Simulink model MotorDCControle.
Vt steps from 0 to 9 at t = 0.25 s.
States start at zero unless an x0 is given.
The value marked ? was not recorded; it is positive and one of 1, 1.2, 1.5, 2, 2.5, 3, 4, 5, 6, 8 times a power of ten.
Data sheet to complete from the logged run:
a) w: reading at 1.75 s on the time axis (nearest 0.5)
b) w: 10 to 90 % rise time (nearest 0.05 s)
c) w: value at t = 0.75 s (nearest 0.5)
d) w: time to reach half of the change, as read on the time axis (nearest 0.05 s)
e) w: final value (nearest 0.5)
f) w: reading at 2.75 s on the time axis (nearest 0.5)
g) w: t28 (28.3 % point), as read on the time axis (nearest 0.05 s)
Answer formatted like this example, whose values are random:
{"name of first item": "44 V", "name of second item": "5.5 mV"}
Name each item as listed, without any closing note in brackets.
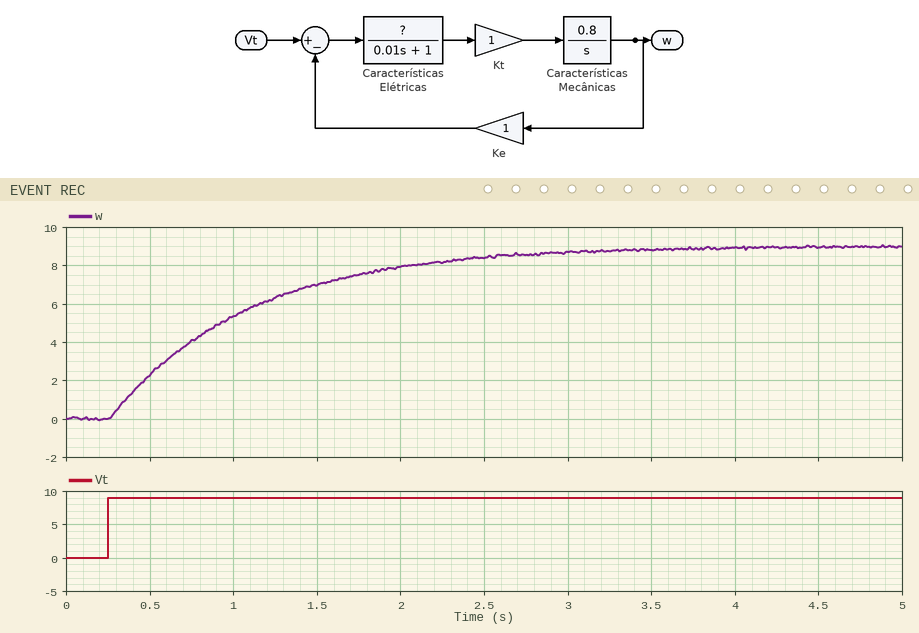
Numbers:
{"w: reading at 1.75 s on the time axis": "7.5", "w: 10 to 90 % rise time": "1.80 s", "w: value at t = 0.75 s": "4.0", "w: time to reach half of the change, as read on the time axis": "0.85 s", "w: final value": "9.0", "w: reading at 2.75 s on the time axis": "8.5", "w: t28 (28.3 % point), as read on the time axis": "0.55 s"}
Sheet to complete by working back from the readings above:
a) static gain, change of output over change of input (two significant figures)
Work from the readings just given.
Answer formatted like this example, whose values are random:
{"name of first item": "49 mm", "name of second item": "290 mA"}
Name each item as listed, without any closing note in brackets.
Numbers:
{"static gain, change of output over change of input": "1.0"}
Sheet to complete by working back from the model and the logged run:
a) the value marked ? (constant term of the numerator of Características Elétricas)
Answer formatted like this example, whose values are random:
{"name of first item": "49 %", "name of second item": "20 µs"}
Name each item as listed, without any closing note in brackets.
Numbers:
{"the value marked ?": "1.5"}
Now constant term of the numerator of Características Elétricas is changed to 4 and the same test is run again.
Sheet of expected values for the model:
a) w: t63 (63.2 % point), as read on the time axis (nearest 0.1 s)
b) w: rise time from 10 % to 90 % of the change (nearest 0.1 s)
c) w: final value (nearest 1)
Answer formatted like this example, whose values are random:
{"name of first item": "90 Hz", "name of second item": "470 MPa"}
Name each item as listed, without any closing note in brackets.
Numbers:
{"w: t63 (63.2 % point), as read on the time axis": "0.6 s", "w: rise time from 10 % to 90 % of the change": "0.7 s", "w: final value": "9"}
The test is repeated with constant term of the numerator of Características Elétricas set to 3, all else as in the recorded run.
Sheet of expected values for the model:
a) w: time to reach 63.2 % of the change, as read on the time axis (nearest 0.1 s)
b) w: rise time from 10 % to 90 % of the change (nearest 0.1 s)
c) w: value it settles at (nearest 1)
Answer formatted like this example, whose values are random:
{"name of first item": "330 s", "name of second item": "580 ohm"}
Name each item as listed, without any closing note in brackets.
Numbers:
{"w: time to reach 63.2 % of the change, as read on the time axis": "0.7 s", "w: rise time from 10 % to 90 % of the change": "0.9 s", "w: value it settles at": "9"}
